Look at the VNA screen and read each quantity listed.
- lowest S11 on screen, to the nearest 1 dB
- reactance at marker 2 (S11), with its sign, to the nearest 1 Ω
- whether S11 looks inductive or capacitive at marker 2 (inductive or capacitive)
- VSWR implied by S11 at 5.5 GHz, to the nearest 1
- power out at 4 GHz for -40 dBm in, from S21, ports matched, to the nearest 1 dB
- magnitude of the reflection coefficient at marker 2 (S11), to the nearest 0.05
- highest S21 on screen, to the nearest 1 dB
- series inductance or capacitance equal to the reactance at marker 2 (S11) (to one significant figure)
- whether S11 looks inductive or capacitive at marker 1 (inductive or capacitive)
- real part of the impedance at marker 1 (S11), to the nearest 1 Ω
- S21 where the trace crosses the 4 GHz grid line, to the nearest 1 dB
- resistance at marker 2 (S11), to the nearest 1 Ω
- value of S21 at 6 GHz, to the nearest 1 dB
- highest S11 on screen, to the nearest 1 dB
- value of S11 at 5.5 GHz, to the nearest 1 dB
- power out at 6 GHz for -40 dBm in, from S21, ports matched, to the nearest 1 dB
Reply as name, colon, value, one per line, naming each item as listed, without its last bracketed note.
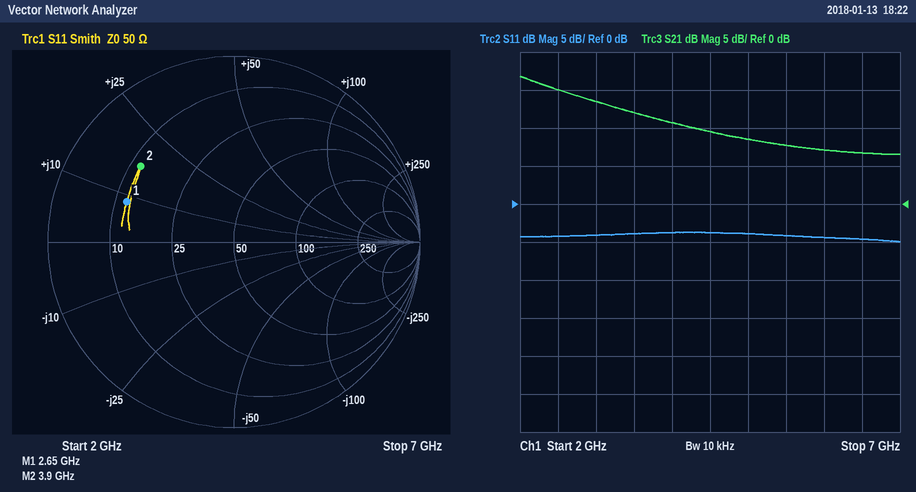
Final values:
lowest S11 on screen, to the nearest 1 dB: -5 dB
reactance at marker 2 (S11), with its sign, to the nearest 1 Ω: +17 Ω
whether S11 looks inductive or capacitive at marker 2: inductive
VSWR implied by S11 at 5.5 GHz, to the nearest 1: 4
power out at 4 GHz for -40 dBm in, from S21, ports matched, to the nearest 1 dB: -29 dBm
magnitude of the reflection coefficient at marker 2 (S11), to the nearest 0.05: 0.65
highest S21 on screen, to the nearest 1 dB: 17 dB
series inductance or capacitance equal to the reactance at marker 2 (S11): 700 pH
whether S11 looks inductive or capacitive at marker 1: inductive
real part of the impedance at marker 1 (S11), to the nearest 1 Ω: 12 Ω
S21 where the trace crosses the 4 GHz grid line, to the nearest 1 dB: 11 dB
resistance at marker 2 (S11), to the nearest 1 Ω: 12 Ω
value of S21 at 6 GHz, to the nearest 1 dB: 7 dB
highest S11 on screen, to the nearest 1 dB: -4 dB
value of S11 at 5.5 GHz, to the nearest 1 dB: -4 dB
power out at 6 GHz for -40 dBm in, from S21, ports matched, to the nearest 1 dB: -33 dBm
